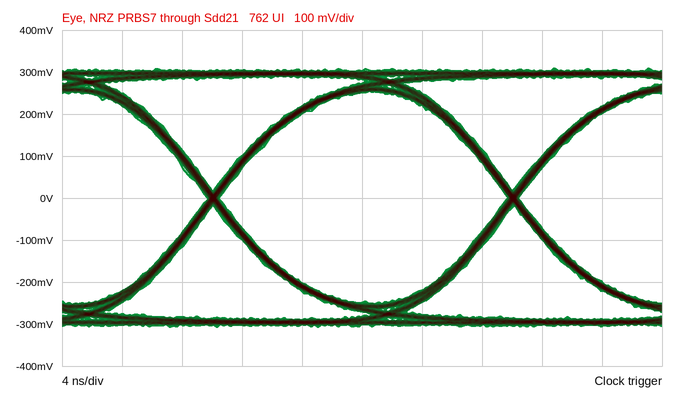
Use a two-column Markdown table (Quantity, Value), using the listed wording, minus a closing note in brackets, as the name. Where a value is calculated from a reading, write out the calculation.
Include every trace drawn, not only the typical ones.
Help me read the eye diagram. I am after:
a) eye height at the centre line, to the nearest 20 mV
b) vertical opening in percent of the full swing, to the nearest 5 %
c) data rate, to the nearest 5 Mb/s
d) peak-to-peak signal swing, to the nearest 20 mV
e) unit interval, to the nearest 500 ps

| Quantity | Value |
|---|---|
| eye height at the centre line, to the nearest 20 mV | 500 mV |
| vertical opening in percent of the full swing, to the nearest 5 % | 500 mV / 620 mV ≈ 80.6 %, so 80 % to the nearest 5 % |
| data rate, to the nearest 5 Mb/s | 50 Mb/s |
| peak-to-peak signal swing, to the nearest 20 mV | 620 mV |
| unit interval, to the nearest 500 ps | 20.0 ns |
